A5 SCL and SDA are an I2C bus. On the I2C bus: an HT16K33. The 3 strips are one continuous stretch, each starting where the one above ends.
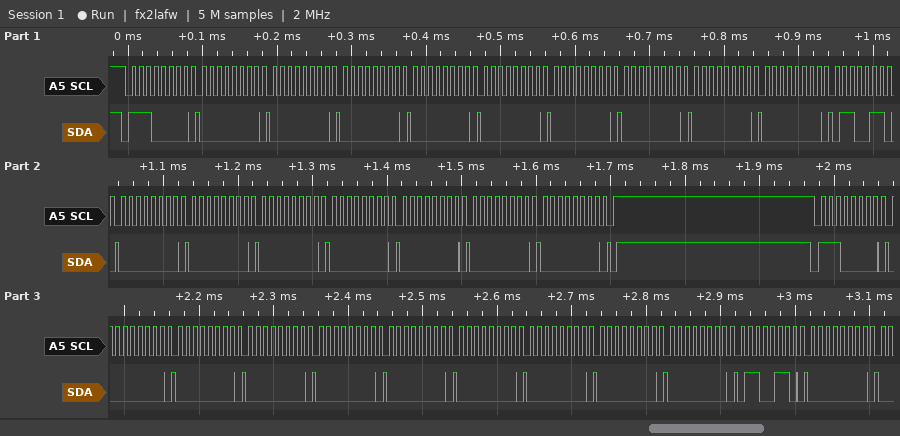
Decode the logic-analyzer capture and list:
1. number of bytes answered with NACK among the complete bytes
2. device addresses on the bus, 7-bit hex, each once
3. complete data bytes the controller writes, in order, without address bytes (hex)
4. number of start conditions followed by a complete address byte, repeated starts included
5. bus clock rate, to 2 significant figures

0
0x70
00 00 00 00 00 00 00 00 00 66 00 00 00 00 00 00 00 00 00 00 00 00 00 00 00 00 66 00
2
100 kHz
